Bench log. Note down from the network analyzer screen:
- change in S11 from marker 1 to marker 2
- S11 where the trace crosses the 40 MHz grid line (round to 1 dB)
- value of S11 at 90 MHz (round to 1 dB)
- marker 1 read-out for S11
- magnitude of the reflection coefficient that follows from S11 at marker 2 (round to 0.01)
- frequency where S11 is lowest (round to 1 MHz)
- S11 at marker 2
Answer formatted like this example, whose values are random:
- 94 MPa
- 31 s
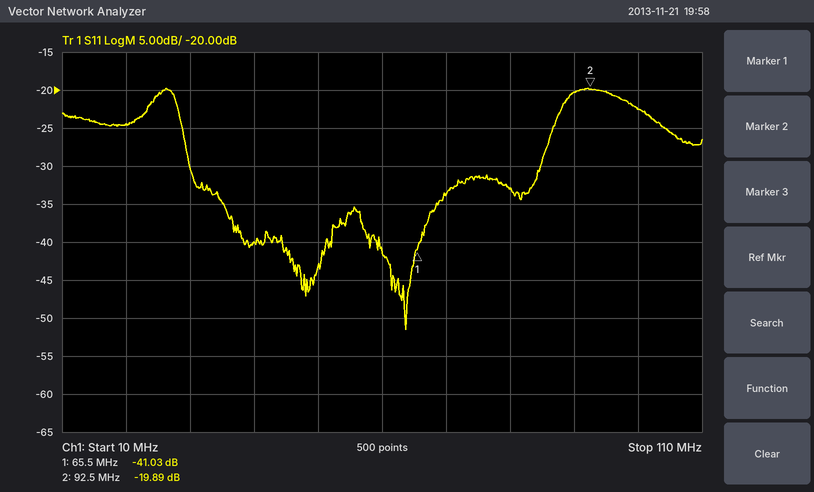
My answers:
- 21.14 dB
- -40 dB
- -20 dB
- -41.03 dB
- 0.10
- 64 MHz
- -19.89 dB
